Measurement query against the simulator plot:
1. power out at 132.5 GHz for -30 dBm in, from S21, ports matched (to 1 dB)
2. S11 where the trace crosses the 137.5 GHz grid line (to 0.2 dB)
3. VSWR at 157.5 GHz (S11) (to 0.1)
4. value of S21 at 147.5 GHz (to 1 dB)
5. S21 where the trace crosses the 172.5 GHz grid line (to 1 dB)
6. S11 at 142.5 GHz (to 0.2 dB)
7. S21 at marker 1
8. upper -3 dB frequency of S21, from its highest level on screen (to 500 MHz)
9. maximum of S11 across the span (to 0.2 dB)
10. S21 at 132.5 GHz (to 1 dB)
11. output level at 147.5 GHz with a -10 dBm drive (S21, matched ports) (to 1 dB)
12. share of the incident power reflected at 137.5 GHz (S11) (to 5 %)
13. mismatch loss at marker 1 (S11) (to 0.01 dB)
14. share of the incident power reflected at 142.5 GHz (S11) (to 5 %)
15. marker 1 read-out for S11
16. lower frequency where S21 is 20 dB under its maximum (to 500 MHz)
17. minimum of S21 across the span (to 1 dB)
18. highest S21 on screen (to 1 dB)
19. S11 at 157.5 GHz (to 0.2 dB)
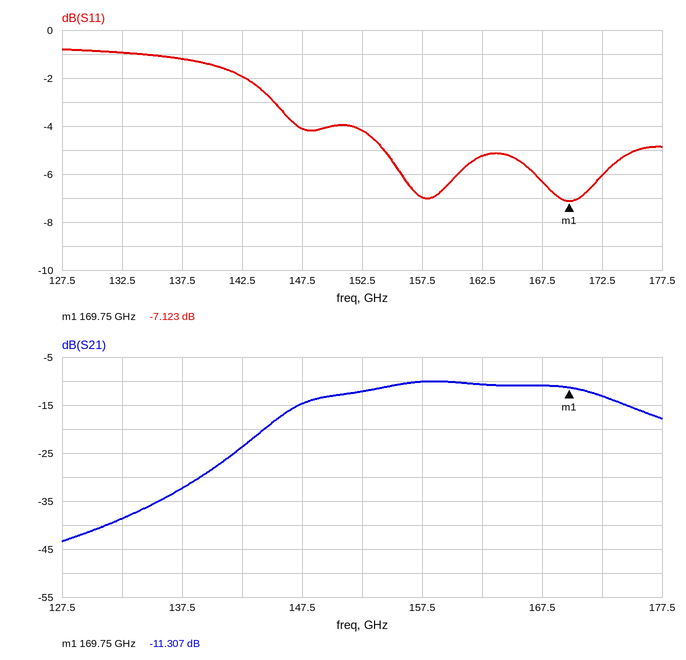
-69 dBm
-1.2 dB
2.6
-15 dB
-13 dB
-2.0 dB
-11.307 dB
172.5 GHz
-0.8 dB
-39 dB
-25 dBm
75 %
0.94 dB
65 %
-7.123 dB
139.0 GHz
-43 dB
-10 dB
-7.0 dB
